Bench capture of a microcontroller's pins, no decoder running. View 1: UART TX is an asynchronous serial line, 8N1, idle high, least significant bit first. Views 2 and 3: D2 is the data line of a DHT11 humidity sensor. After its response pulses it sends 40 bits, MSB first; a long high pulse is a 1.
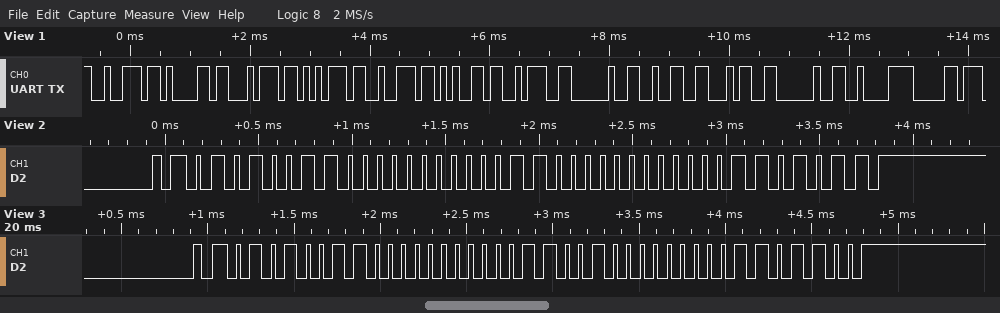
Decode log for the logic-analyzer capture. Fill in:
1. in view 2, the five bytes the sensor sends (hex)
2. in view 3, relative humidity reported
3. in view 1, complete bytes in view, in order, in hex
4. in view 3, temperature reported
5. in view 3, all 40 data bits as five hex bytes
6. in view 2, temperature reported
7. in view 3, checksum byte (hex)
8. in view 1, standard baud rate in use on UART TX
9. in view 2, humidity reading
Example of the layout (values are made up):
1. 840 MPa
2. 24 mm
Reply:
1. 53 00 18 00 6B
2. 83 %
3. 72 61 74 75 72 65 3A 20 32 34 20 C2 B0
4. 25.0 °C
5. 53 00 19 00 6C
6. 24.0 °C
7. 0x6C
8. 9600 baud
9. 83 %
